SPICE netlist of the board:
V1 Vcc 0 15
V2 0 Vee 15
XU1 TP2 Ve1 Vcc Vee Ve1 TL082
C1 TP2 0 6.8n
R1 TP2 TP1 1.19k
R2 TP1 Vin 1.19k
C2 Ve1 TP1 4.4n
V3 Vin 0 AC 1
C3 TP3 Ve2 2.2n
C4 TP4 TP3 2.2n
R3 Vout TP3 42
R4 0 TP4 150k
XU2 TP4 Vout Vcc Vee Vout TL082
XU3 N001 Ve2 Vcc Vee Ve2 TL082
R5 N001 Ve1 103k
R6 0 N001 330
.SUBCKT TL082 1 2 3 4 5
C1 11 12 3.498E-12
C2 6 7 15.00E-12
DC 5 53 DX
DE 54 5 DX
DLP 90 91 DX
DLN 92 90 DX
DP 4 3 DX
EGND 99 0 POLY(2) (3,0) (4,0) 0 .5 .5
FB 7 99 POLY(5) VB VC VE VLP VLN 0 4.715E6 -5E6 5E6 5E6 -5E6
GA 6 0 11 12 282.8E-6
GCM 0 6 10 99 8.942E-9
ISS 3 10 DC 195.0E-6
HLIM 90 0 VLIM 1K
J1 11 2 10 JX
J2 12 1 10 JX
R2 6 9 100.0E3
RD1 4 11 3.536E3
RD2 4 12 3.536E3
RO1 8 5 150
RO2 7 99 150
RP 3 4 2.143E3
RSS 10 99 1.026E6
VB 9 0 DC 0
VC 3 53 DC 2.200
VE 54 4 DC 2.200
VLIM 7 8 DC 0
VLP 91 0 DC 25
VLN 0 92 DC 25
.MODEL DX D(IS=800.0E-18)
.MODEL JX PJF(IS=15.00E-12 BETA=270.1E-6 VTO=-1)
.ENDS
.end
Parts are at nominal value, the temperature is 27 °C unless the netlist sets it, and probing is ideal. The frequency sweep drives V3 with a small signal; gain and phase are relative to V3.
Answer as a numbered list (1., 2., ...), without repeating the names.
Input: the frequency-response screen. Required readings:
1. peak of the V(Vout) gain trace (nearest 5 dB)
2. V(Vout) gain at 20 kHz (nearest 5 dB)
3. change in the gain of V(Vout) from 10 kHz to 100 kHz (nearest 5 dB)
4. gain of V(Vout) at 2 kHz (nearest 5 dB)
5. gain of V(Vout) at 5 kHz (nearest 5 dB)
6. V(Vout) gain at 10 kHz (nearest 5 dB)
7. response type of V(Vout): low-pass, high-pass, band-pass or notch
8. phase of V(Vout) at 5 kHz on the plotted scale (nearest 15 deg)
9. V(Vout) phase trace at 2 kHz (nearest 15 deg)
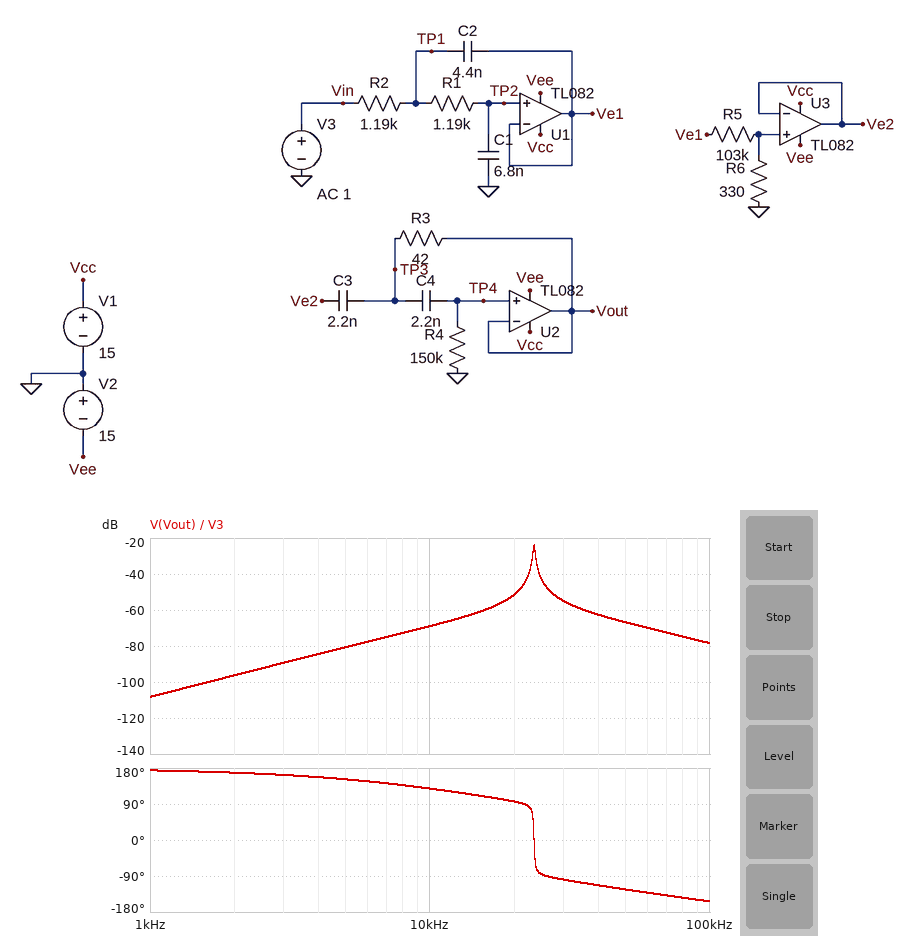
1. -25 dB
2. -50 dB
3. -10 dB
4. -95 dB
5. -80 dB
6. -70 dB
7. band-pass
8. 150 deg
9. 165 deg
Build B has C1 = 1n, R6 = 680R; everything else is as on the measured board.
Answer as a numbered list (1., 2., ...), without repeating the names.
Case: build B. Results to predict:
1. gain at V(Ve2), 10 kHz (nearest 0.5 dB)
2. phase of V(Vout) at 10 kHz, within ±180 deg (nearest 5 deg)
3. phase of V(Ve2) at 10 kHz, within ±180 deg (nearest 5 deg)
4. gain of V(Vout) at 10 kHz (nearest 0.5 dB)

1. -43.5 dB
2. 170 deg
3. -10 deg
4. -60.0 dB
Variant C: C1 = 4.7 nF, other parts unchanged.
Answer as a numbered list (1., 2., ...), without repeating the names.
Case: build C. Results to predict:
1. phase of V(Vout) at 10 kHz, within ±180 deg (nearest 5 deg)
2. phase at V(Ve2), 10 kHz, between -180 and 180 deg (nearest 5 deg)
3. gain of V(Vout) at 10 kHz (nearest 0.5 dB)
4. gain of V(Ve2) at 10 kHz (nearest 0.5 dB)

1. 140 deg
2. -40 deg
3. -67.5 dB
4. -51.0 dB
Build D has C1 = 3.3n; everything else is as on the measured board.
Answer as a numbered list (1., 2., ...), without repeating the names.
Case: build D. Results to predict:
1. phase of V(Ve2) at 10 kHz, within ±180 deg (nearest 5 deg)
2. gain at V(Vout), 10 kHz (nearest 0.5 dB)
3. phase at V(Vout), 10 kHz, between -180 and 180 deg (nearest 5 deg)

1. -30 deg
2. -67.0 dB
3. 150 deg
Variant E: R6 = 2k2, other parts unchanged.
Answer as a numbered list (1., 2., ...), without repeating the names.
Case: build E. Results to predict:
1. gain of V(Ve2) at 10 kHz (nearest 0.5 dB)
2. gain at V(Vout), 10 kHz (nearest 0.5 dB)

1. -36.0 dB
2. -52.5 dB
